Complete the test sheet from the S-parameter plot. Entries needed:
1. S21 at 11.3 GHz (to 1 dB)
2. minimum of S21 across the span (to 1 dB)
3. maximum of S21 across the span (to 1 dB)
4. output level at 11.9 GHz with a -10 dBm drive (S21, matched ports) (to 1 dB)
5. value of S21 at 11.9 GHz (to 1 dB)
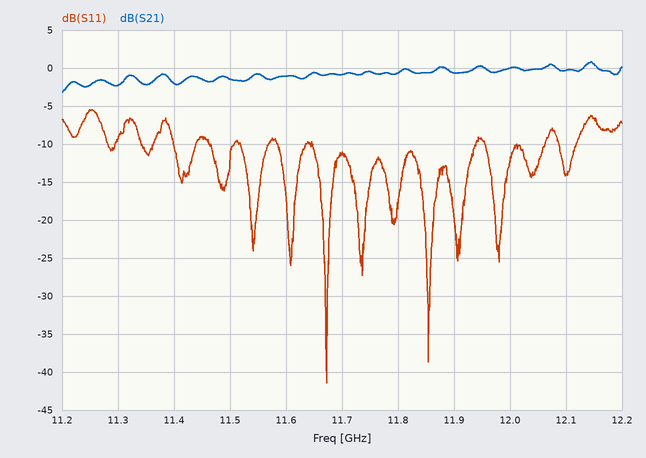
-2 dB
-3 dB
1 dB
-11 dBm
-1 dB
